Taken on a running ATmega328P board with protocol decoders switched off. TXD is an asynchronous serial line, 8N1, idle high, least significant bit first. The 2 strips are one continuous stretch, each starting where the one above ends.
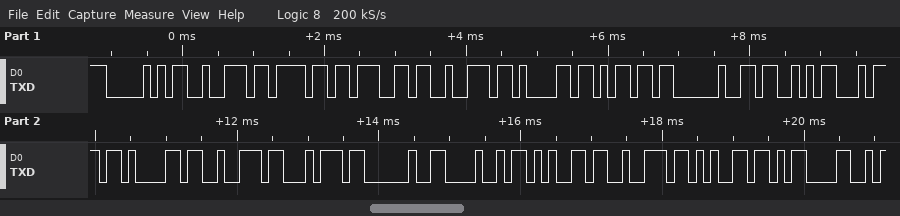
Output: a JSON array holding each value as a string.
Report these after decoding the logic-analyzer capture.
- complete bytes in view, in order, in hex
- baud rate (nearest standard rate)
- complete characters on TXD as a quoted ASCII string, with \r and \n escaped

["50 72 6F 67 72 61 6D 20 53 74 61 72 74 20 48 65 72 65 0D", "9600 baud", "\"Program Start Here\\r\""]
